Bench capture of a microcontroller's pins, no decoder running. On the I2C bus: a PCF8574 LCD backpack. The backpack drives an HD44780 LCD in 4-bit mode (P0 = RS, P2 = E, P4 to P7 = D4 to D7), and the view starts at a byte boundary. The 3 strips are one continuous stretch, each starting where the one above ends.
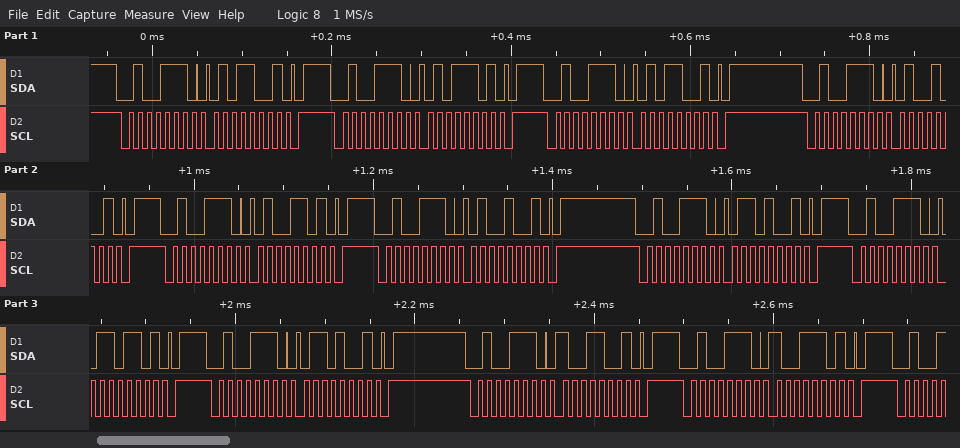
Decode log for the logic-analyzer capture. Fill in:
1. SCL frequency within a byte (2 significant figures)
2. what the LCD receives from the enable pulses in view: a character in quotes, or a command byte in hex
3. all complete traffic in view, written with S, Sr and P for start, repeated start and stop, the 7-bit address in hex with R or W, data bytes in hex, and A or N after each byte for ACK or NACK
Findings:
100 kHz
'T'
S 27W A 59 A P S 27W A 5D A P S 27W A 59 A P S 27W A 49 A P S 27W A 4D A P S 27W A 49 A P S 27W A 69 A P S 27W A 6D A P S 27W A 69 A P S 27W A 99 A P S 27W A 9D A P
